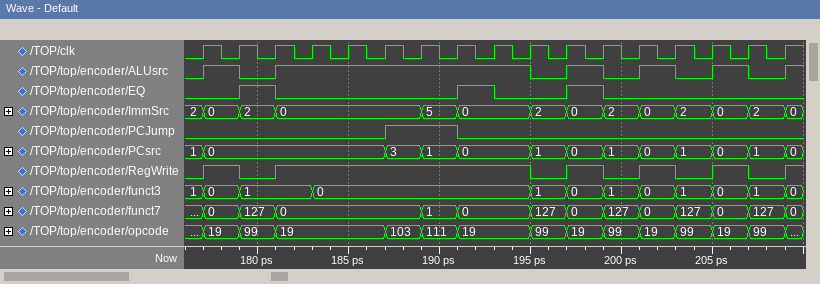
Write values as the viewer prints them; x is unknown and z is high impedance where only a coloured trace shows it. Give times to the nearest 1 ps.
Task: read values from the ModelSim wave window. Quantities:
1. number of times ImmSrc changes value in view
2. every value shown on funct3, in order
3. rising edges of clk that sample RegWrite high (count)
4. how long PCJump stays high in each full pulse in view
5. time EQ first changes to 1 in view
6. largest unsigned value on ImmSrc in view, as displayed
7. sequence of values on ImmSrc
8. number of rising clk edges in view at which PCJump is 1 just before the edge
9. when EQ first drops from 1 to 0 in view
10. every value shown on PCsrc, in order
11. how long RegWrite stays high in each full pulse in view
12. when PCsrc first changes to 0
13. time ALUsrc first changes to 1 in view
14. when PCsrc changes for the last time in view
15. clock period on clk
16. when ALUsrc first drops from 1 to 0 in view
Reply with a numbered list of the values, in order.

1. 13
2. 1, 0, 1, 0, 1, 0, 1, 0, 1, 0, 1, 0
3. 11
4. 4 ps
5. 179 ps
6. 5
7. 2, 0, 2, 0, 5, 0, 2, 0, 2, 0, 2, 0, 2, 0
8. 2
9. 181 ps
10. 1, 0, 3, 1, 0, 1, 0, 1, 0, 1, 0, 1, 0
11. 2 ps, 14 ps, 2 ps, 2 ps, 2 ps
12. 177 ps
13. 177 ps
14. 209 ps
15. 2 ps
16. 179 ps
